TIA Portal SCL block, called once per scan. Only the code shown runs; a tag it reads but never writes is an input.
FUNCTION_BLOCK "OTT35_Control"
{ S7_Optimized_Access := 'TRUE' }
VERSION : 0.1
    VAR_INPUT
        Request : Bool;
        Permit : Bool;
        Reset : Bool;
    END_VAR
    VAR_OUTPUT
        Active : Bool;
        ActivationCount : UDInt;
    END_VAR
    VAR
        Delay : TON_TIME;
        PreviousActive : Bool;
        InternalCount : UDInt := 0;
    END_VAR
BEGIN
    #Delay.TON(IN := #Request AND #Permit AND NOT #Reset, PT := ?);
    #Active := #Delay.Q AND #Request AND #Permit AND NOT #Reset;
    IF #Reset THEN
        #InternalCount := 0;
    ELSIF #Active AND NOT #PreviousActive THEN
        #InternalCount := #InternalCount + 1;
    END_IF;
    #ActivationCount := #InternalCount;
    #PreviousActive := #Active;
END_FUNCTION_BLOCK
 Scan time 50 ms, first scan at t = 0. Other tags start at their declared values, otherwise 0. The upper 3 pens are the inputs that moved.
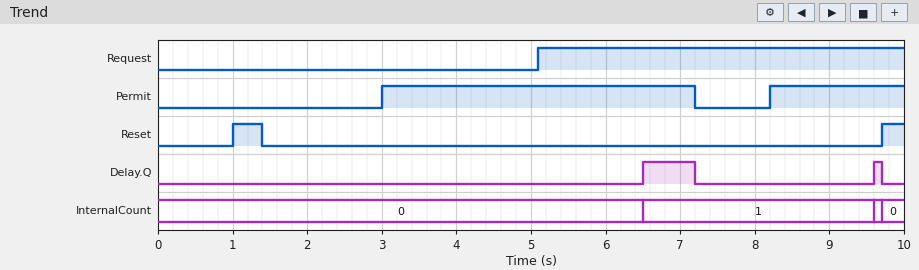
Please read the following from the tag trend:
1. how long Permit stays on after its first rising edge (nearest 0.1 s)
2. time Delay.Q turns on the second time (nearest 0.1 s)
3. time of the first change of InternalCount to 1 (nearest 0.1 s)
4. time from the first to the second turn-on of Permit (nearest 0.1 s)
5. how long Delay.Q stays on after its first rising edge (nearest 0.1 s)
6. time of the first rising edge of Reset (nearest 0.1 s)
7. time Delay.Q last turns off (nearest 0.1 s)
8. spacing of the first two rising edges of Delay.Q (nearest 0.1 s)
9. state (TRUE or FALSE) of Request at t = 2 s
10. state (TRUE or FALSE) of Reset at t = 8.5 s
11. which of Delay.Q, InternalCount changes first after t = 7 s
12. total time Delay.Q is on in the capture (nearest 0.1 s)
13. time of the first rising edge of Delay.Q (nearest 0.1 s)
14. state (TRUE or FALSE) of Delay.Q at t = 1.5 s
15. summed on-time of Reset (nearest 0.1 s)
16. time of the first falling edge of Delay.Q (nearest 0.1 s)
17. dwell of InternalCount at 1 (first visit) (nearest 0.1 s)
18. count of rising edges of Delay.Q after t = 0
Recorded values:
4.2 s
9.6 s
6.5 s
5.2 s
0.7 s
1.0 s
9.7 s
3.1 s
FALSE
FALSE
Delay.Q
0.8 s
6.5 s
FALSE
0.7 s
7.2 s
3.1 s
2
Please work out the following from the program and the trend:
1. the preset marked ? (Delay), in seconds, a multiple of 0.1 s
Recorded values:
1.4 s
